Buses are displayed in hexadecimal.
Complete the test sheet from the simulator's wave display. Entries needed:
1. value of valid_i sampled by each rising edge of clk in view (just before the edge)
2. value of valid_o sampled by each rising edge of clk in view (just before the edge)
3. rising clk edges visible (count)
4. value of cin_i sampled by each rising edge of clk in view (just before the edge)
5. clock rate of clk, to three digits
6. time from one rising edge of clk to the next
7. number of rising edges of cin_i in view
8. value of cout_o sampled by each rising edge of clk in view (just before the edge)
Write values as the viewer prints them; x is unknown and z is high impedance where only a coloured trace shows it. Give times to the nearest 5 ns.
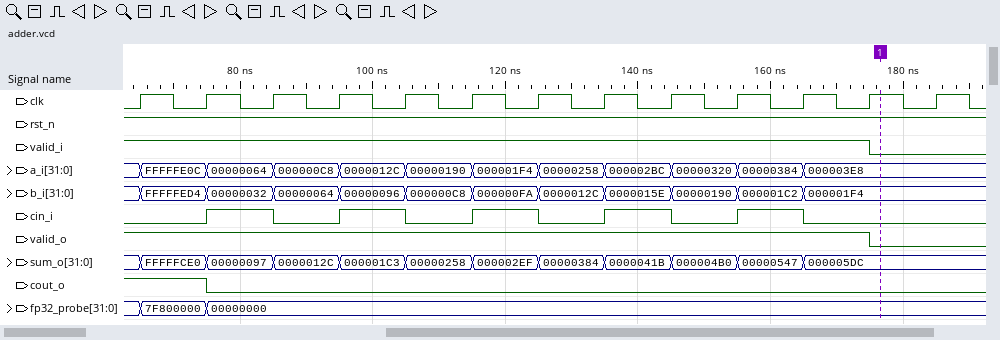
1 1 1 1 1 1 1 1 1 1 1 1 0
1 1 1 1 1 1 1 1 1 1 1 1 0
13
0 0 1 0 1 0 1 0 1 0 1 0 0
100 MHz
10 ns
5
1 1 0 0 0 0 0 0 0 0 0 0 0
